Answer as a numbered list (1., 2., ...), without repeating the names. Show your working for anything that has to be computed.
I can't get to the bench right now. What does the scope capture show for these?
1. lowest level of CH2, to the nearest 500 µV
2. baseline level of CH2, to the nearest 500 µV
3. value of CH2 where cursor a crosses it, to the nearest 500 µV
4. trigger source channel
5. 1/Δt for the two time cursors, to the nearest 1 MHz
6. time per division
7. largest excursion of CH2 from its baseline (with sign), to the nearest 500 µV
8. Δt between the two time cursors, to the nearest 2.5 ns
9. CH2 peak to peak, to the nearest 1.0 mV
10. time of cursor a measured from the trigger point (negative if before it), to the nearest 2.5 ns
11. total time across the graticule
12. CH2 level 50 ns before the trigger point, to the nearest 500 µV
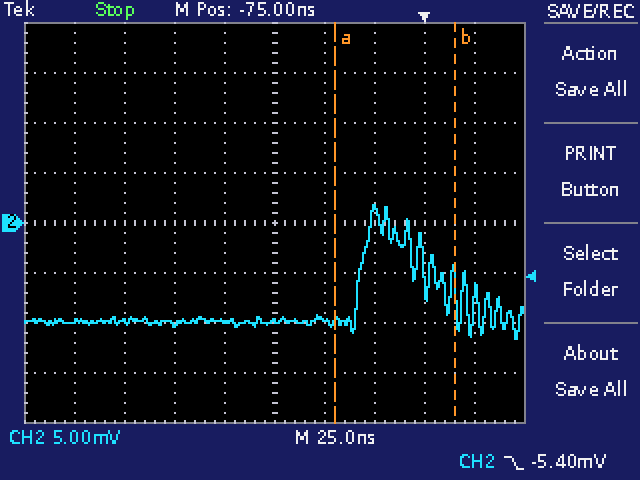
1. -11.5 mV
2. -10.0 mV
3. -10.0 mV
4. CH2
5. 1 / 60.0 ns ≈ 17 MHz
6. 25 ns
7. +11.5 mV
8. 60.0 ns
9. 13.0 mV
10. -45.0 ns
11. 250 ns
12. -9.5 mV
